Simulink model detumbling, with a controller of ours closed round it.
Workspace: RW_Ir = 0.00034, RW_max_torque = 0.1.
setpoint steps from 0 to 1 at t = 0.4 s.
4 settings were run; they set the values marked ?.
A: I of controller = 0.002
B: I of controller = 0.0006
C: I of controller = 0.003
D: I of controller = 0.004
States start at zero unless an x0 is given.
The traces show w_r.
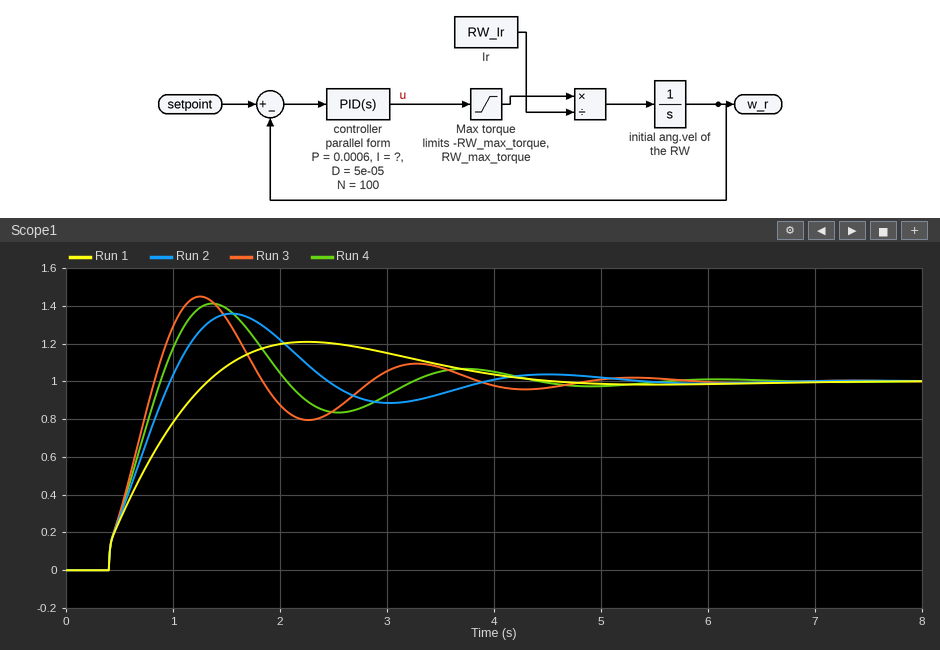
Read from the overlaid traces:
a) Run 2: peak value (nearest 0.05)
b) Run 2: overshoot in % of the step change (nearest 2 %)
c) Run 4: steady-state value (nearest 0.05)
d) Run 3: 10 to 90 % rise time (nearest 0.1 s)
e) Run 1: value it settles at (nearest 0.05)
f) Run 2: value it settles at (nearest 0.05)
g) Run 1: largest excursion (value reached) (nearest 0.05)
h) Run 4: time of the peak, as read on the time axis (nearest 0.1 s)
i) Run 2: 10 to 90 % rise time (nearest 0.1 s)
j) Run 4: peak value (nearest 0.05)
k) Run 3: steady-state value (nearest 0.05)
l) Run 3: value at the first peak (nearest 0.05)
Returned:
1.35
36 %
1.00
0.4 s
1.00
1.00
1.20
1.4 s
0.5 s
1.40
1.00
1.45
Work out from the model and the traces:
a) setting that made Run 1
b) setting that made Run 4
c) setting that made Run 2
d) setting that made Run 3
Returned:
B
C
A
D
